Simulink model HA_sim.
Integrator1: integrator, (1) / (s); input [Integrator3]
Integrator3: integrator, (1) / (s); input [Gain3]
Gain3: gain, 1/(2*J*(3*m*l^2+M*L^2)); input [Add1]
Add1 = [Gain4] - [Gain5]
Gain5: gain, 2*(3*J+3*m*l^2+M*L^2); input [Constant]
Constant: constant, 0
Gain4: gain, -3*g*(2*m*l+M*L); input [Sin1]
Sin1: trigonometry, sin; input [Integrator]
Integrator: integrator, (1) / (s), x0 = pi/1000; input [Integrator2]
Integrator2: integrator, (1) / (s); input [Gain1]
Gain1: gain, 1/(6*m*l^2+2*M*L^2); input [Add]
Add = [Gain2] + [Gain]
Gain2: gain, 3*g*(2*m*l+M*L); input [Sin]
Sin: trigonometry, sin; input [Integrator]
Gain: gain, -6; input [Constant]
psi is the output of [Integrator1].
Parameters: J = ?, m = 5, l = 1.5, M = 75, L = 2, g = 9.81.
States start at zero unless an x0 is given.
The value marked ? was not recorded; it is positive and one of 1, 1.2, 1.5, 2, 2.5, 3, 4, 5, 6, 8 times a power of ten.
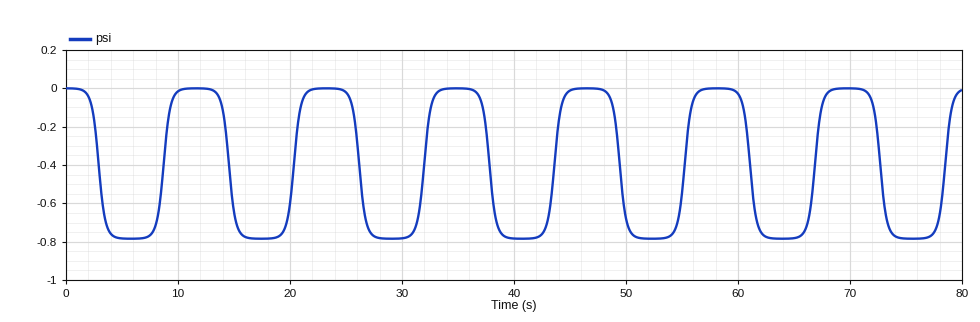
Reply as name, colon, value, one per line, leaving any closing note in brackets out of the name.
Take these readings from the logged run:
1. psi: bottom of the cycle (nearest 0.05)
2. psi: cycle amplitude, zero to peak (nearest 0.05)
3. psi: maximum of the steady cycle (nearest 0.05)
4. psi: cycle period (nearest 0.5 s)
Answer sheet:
psi: bottom of the cycle: -0.80
psi: cycle amplitude, zero to peak: 0.40
psi: maximum of the steady cycle: 0.00
psi: cycle period: 11.5 s
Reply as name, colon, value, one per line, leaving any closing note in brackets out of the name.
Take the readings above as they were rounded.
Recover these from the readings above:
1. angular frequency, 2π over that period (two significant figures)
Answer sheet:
angular frequency, 2π over that period: 0.55 rad/s
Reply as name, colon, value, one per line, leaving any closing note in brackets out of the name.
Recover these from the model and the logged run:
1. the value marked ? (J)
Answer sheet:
the value marked ?: 8
